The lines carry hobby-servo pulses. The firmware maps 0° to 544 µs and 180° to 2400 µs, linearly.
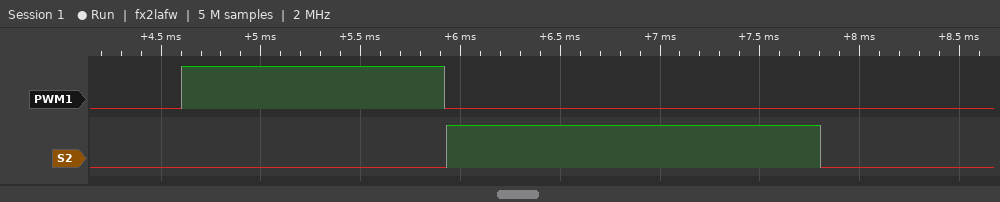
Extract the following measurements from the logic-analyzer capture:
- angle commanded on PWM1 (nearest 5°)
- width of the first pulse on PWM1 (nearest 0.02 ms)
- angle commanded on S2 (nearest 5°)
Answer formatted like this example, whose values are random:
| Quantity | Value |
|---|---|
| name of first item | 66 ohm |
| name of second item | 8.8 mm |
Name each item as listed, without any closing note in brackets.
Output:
| Quantity | Value |
|---|---|
| angle commanded on PWM1 | 75° |
| width of the first pulse on PWM1 | 1.32 ms |
| angle commanded on S2 | 130° |
